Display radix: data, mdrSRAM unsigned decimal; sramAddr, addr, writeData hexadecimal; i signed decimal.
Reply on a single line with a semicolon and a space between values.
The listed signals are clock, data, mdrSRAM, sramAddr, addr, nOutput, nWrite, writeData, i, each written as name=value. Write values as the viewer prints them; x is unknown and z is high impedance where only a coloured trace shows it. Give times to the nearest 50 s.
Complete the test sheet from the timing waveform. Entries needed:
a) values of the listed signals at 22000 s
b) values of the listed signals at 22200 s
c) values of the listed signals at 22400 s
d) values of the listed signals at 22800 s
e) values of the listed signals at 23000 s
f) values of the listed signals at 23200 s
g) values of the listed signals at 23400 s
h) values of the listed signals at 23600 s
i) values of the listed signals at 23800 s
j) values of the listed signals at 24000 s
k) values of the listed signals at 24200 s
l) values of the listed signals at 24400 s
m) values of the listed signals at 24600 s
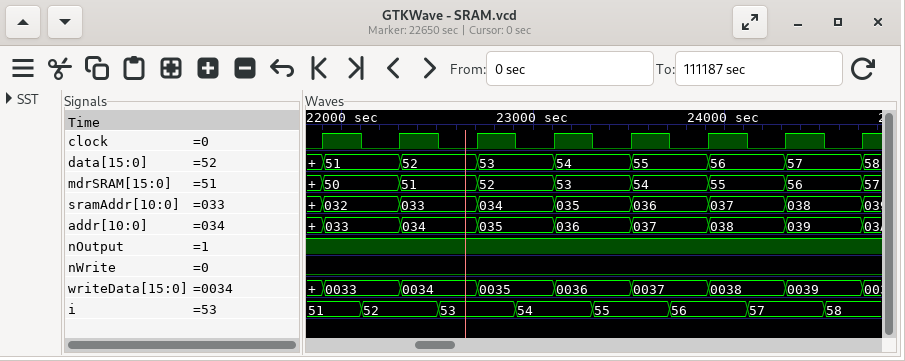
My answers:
clock=1, data=51, mdrSRAM=50, sramAddr=032, addr=033, nOutput=1, nWrite=0, writeData=0033, i=51; clock=0, data=51, mdrSRAM=50, sramAddr=032, addr=033, nOutput=1, nWrite=0, writeData=0033, i=52; clock=1, data=52, mdrSRAM=51, sramAddr=033, addr=034, nOutput=1, nWrite=0, writeData=0034, i=52; clock=1, data=53, mdrSRAM=52, sramAddr=034, addr=035, nOutput=1, nWrite=0, writeData=0035, i=53; clock=0, data=53, mdrSRAM=52, sramAddr=034, addr=035, nOutput=1, nWrite=0, writeData=0035, i=54; clock=1, data=54, mdrSRAM=53, sramAddr=035, addr=036, nOutput=1, nWrite=0, writeData=0036, i=54; clock=0, data=54, mdrSRAM=53, sramAddr=035, addr=036, nOutput=1, nWrite=0, writeData=0036, i=55; clock=1, data=55, mdrSRAM=54, sramAddr=036, addr=037, nOutput=1, nWrite=0, writeData=0037, i=55; clock=0, data=55, mdrSRAM=54, sramAddr=036, addr=037, nOutput=1, nWrite=0, writeData=0037, i=56; clock=1, data=56, mdrSRAM=55, sramAddr=037, addr=038, nOutput=1, nWrite=0, writeData=0038, i=56; clock=0, data=56, mdrSRAM=55, sramAddr=037, addr=038, nOutput=1, nWrite=0, writeData=0038, i=57; clock=1, data=57, mdrSRAM=56, sramAddr=038, addr=039, nOutput=1, nWrite=0, writeData=0039, i=57; clock=0, data=57, mdrSRAM=56, sramAddr=038, addr=039, nOutput=1, nWrite=0, writeData=0039, i=58
